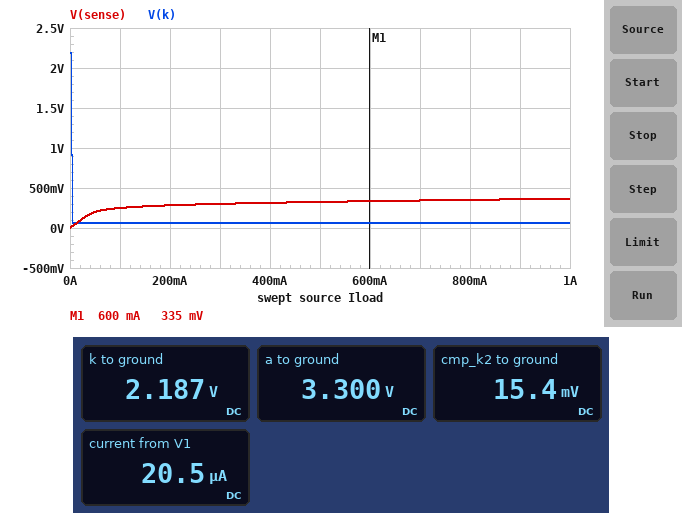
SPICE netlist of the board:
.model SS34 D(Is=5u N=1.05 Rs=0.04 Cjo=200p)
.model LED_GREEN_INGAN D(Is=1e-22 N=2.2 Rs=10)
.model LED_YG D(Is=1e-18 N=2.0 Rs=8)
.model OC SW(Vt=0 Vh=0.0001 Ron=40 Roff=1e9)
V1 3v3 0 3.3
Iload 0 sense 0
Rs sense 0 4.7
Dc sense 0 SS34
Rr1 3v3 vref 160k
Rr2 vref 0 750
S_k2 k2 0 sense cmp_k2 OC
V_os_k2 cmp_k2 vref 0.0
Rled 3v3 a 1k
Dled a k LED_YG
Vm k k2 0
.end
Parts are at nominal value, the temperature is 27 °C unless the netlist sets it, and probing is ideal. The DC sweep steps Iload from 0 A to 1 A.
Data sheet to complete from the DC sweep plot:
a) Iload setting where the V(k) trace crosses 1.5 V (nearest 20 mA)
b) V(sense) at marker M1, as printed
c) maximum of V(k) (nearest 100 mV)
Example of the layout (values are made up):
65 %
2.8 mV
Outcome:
0 A
335 mV
2.2 V
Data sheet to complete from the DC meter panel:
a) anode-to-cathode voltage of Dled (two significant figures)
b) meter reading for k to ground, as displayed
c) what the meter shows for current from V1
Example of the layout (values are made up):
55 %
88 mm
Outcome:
1.1 V
2.187 V
20.5 µA
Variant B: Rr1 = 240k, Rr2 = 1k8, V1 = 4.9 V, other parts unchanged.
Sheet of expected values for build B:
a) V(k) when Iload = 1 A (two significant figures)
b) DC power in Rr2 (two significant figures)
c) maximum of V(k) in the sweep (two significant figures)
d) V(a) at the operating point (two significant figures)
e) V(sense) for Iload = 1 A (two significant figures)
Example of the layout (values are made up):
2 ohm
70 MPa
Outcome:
120 mV
740 nW
3.8 V
4.9 V
370 mV
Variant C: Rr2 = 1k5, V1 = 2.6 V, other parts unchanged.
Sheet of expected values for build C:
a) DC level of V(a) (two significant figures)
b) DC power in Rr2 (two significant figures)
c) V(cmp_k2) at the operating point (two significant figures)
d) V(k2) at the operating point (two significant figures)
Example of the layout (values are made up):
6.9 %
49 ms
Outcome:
2.6 V
390 nW
24 mV
1.5 V
